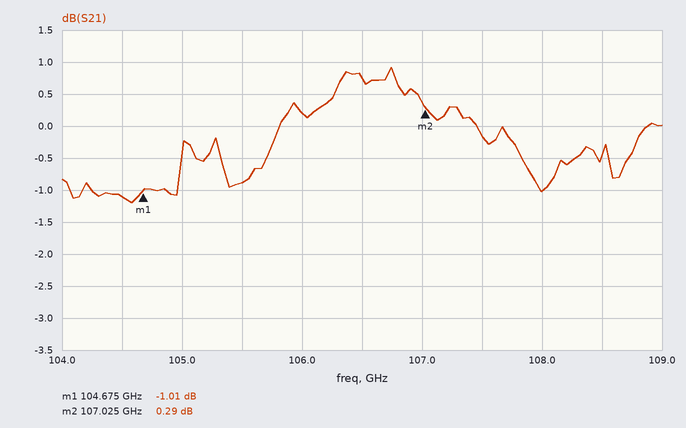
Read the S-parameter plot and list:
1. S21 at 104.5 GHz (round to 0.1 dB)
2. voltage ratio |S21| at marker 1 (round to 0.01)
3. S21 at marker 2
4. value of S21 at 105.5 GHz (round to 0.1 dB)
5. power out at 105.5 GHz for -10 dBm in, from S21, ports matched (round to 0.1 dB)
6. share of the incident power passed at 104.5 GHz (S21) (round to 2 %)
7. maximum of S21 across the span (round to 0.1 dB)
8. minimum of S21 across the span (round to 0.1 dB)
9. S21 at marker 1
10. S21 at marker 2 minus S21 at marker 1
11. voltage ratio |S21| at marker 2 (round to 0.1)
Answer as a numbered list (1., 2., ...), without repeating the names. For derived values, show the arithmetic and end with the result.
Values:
1. -1.1 dB
2. 10^(-1.01/20) ≈ 0.89
3. 0.29 dB
4. -0.9 dB
5. -10 dBm + (-0.9 dB) = -10.9 dBm
6. 10^(-1.1/10) ≈ 78 %
7. 0.9 dB
8. -1.2 dB
9. -1.01 dB
10. 0.29 − (-1.01) = 1.30 dB
11. 10^(0.29/20) ≈ 1.0
